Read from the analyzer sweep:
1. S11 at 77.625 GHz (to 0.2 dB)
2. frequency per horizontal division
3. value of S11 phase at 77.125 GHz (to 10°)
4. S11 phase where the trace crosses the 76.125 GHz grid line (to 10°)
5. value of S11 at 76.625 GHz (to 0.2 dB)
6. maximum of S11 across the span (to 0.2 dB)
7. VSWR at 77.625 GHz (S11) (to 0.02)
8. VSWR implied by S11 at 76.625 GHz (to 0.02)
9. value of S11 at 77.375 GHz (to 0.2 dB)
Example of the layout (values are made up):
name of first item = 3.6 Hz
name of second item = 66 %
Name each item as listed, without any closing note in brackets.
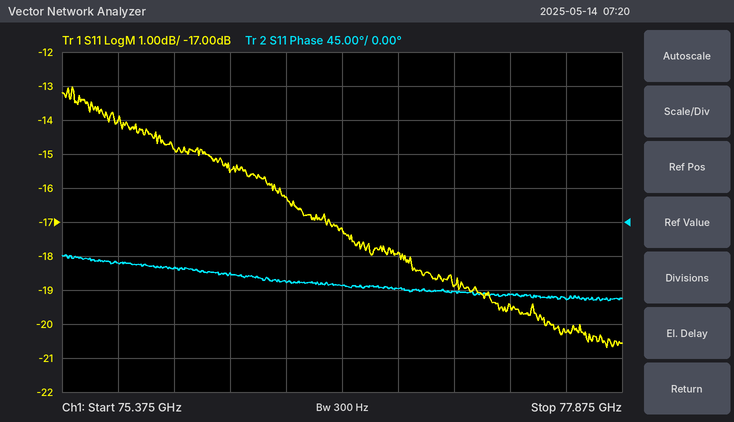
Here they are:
S11 at 77.625 GHz = -20.2 dB
frequency per horizontal division = 250 MHz
value of S11 phase at 77.125 GHz = -90°
S11 phase where the trace crosses the 76.125 GHz grid line = -70°
value of S11 at 76.625 GHz = -17.2 dB
maximum of S11 across the span = -13.0 dB
VSWR at 77.625 GHz (S11) = 1.22
VSWR implied by S11 at 76.625 GHz = 1.32
value of S11 at 77.375 GHz = -19.4 dB
